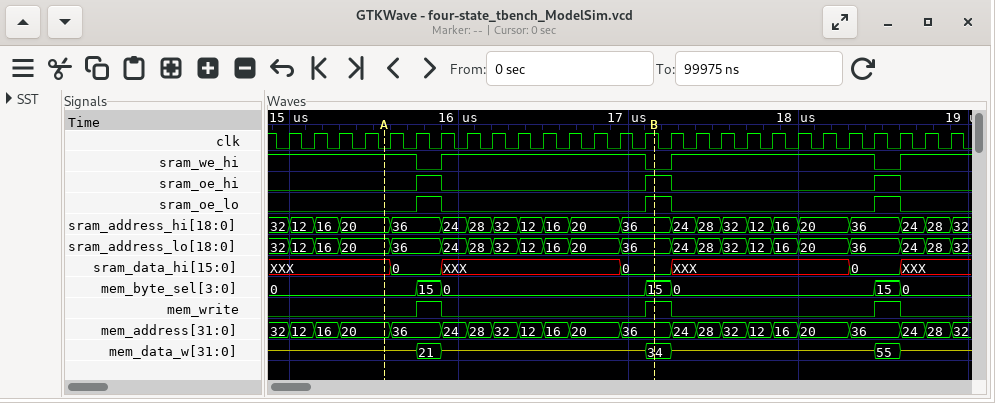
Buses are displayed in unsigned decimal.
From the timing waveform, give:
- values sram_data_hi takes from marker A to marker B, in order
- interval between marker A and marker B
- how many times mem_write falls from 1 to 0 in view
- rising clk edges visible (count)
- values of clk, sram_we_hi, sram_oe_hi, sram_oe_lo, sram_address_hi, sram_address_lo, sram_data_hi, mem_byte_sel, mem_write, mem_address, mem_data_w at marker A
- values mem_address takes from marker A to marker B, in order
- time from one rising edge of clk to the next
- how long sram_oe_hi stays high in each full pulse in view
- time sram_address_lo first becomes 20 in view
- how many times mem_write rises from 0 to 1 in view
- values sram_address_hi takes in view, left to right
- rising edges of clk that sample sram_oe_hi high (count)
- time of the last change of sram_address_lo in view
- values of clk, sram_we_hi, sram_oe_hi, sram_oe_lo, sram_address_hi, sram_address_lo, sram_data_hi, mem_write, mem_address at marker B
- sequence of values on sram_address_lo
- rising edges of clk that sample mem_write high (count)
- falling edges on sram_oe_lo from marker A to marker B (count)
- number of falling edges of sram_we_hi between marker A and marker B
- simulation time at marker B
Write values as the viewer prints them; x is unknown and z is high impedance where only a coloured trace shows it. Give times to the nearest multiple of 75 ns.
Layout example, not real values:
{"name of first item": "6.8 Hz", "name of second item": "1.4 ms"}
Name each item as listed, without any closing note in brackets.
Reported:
{"values sram_data_hi takes from marker A to marker B, in order": "XXX, 0, XXX, 0", "interval between marker A and marker B": "1575 ns", "how many times mem_write falls from 1 to 0 in view": "3", "rising clk edges visible": "27", "values of clk, sram_we_hi, sram_oe_hi, sram_oe_lo, sram_address_hi, sram_address_lo, sram_data_hi, mem_byte_sel, mem_write, mem_address, mem_data_w at marker A": "clk=0, sram_we_hi=1, sram_oe_hi=0, sram_oe_lo=0, sram_address_hi=20, sram_address_lo=20, sram_data_hi=XXX, mem_byte_sel=0, mem_write=0, mem_address=20, mem_data_w=z", "values mem_address takes from marker A to marker B, in order": "20, 36, 24, 28, 32, 12, 16, 20, 36", "time from one rising edge of clk to the next": "150 ns", "how long sram_oe_hi stays high in each full pulse in view": "150 ns, 150 ns, 150 ns", "time sram_address_lo first becomes 20 in view": "15300 ns", "how many times mem_write rises from 0 to 1 in view": "3", "values sram_address_hi takes in view, left to right": "32, 12, 16, 20, 36, 24, 28, 32, 12, 16, 20, 36, 24, 28, 32, 12, 16, 20, 36, 24, 28, 32", "rising edges of clk that sample sram_oe_hi high": "3", "time of the last change of sram_address_lo in view": "18900 ns", "values of clk, sram_we_hi, sram_oe_hi, sram_oe_lo, sram_address_hi, sram_address_lo, sram_data_hi, mem_write, mem_address at marker B": "clk=1, sram_we_hi=0, sram_oe_hi=1, sram_oe_lo=1, sram_address_hi=36, sram_address_lo=36, sram_data_hi=0, mem_write=1, mem_address=36", "sequence of values on sram_address_lo": "32, 12, 16, 20, 36, 24, 28, 32, 12, 16, 20, 36, 24, 28, 32, 12, 16, 20, 36, 24, 28, 32", "rising edges of clk that sample mem_write high": "3", "falling edges on sram_oe_lo from marker A to marker B": "1", "number of falling edges of sram_we_hi between marker A and marker B": "2", "simulation time at marker B": "17175 ns"}
